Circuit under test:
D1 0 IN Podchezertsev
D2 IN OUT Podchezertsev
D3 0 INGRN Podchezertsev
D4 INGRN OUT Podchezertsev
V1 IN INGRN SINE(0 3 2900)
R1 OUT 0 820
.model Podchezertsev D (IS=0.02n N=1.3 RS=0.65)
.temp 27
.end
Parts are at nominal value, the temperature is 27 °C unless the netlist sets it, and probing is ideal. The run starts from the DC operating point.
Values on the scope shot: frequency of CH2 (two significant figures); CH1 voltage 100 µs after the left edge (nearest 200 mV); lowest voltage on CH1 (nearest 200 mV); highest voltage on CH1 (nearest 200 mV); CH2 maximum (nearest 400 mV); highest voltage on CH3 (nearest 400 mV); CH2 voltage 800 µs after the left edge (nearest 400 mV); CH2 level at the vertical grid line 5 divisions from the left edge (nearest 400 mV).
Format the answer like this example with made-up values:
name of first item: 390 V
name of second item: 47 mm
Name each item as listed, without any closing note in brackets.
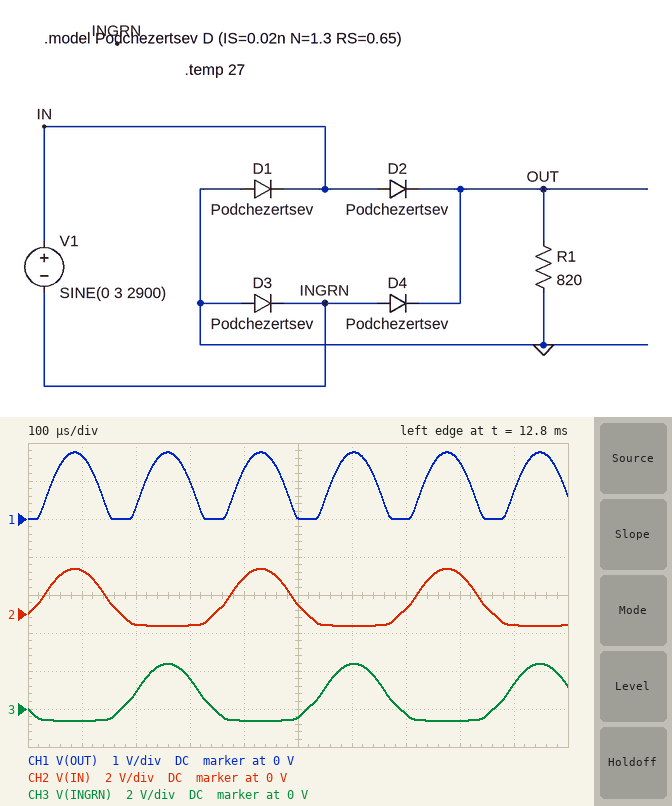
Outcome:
frequency of CH2: 2.9 kHz
CH1 voltage 100 µs after the left edge: 1.6 V
lowest voltage on CH1: 0 V
highest voltage on CH1: 1.8 V
CH2 maximum: 2.4 V
highest voltage on CH3: 2.4 V
CH2 voltage 800 µs after the left edge: 2.0 V
CH2 level at the vertical grid line 5 divisions from the left edge: 400 mV
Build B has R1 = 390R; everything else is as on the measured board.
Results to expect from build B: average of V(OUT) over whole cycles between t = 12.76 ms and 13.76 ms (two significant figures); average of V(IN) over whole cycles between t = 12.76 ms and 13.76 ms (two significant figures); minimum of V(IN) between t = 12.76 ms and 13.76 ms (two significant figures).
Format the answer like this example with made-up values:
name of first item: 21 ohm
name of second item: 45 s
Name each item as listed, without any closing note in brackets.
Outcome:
average of V(OUT) over whole cycles between t = 12.76 ms and 13.76 ms: 830 mV
average of V(IN) over whole cycles between t = 12.76 ms and 13.76 ms: 410 mV
minimum of V(IN) between t = 12.76 ms and 13.76 ms: -650 mV
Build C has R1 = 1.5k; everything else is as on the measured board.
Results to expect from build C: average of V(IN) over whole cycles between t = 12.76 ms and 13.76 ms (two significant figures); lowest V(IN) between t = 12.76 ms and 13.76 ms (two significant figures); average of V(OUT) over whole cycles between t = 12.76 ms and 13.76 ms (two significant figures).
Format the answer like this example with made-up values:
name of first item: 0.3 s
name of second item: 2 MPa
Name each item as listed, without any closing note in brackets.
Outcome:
average of V(IN) over whole cycles between t = 12.76 ms and 13.76 ms: 450 mV
lowest V(IN) between t = 12.76 ms and 13.76 ms: -600 mV
average of V(OUT) over whole cycles between t = 12.76 ms and 13.76 ms: 890 mV
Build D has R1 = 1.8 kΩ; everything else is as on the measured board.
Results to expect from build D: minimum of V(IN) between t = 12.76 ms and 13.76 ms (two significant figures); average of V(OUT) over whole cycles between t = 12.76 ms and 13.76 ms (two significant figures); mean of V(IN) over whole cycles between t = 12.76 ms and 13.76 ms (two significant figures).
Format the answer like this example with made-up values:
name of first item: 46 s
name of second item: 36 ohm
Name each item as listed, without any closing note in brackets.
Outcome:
minimum of V(IN) between t = 12.76 ms and 13.76 ms: -600 mV
average of V(OUT) over whole cycles between t = 12.76 ms and 13.76 ms: 900 mV
mean of V(IN) over whole cycles between t = 12.76 ms and 13.76 ms: 450 mV
